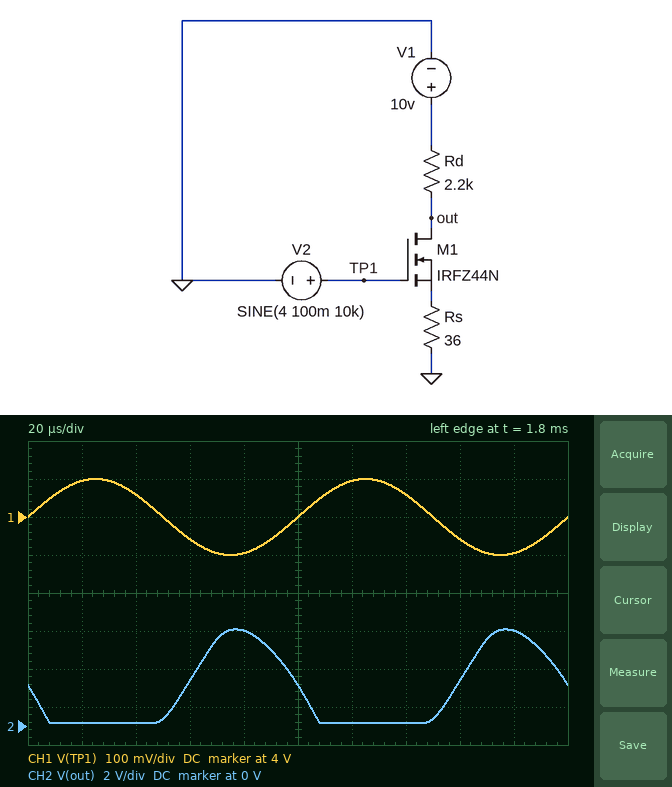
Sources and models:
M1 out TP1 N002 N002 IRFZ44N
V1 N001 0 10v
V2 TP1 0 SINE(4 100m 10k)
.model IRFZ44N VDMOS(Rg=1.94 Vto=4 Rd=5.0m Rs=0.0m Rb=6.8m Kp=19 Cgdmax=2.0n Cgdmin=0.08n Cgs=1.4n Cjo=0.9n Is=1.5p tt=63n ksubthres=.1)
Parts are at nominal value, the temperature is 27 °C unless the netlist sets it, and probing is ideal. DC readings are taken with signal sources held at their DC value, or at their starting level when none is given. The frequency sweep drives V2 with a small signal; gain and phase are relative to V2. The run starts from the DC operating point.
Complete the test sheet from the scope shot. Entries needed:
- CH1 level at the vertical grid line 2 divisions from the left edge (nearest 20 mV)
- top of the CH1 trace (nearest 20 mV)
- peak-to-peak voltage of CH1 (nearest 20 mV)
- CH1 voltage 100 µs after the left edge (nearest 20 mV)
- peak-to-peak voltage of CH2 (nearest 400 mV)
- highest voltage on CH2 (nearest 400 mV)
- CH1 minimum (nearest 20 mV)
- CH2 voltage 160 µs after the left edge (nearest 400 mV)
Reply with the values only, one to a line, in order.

4.06 V
4.10 V
200 mV
4.00 V
4.8 V
5.2 V
3.90 V
2.4 V
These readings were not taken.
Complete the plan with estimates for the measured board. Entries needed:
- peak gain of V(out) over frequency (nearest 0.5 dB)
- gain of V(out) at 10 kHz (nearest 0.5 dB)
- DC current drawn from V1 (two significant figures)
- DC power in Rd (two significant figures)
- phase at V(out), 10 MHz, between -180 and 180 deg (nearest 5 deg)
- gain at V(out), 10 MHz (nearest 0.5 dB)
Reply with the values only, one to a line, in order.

33.0 dB
32.5 dB
4.1 mA
37 mW
5 deg
0 dB
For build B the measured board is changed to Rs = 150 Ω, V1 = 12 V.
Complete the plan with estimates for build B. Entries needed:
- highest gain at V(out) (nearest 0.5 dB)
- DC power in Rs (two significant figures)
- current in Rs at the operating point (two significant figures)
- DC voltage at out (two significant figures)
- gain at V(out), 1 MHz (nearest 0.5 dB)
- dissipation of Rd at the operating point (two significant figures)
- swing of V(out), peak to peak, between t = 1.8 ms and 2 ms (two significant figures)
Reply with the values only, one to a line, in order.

21.5 dB
280 µW
1.4 mA
9.0 V
10.0 dB
4.1 mW
2.3 V
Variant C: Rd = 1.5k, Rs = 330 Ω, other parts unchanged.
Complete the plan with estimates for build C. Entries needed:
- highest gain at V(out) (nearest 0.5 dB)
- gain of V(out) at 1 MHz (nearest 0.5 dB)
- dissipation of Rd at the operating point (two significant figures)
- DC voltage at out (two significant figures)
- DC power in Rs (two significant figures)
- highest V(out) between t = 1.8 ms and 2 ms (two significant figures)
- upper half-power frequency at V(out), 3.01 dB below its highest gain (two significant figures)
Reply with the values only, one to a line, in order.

11.5 dB
5.5 dB
790 µW
8.9 V
170 µW
9.3 V
540 kHz
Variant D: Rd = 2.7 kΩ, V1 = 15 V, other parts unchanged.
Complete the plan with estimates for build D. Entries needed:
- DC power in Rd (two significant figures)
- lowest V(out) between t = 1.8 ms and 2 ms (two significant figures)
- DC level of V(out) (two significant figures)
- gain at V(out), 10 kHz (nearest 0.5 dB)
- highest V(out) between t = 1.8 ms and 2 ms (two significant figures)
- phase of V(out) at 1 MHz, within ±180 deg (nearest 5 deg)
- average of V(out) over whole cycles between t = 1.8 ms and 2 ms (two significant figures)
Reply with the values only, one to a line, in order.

45 mW
210 mV
4.0 V
34.5 dB
9.0 V
65 deg
4.1 V
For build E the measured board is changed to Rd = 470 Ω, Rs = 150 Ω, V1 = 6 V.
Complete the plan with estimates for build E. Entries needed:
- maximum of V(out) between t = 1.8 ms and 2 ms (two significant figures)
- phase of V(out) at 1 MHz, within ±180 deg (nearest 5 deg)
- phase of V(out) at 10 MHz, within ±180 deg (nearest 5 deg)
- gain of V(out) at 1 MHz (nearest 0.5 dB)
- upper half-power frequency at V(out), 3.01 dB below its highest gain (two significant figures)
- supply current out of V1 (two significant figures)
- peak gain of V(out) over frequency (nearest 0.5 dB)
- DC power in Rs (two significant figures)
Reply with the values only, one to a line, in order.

5.6 V
70 deg
5 deg
4.5 dB
860 kHz
1.4 mA
8.0 dB
280 µW
